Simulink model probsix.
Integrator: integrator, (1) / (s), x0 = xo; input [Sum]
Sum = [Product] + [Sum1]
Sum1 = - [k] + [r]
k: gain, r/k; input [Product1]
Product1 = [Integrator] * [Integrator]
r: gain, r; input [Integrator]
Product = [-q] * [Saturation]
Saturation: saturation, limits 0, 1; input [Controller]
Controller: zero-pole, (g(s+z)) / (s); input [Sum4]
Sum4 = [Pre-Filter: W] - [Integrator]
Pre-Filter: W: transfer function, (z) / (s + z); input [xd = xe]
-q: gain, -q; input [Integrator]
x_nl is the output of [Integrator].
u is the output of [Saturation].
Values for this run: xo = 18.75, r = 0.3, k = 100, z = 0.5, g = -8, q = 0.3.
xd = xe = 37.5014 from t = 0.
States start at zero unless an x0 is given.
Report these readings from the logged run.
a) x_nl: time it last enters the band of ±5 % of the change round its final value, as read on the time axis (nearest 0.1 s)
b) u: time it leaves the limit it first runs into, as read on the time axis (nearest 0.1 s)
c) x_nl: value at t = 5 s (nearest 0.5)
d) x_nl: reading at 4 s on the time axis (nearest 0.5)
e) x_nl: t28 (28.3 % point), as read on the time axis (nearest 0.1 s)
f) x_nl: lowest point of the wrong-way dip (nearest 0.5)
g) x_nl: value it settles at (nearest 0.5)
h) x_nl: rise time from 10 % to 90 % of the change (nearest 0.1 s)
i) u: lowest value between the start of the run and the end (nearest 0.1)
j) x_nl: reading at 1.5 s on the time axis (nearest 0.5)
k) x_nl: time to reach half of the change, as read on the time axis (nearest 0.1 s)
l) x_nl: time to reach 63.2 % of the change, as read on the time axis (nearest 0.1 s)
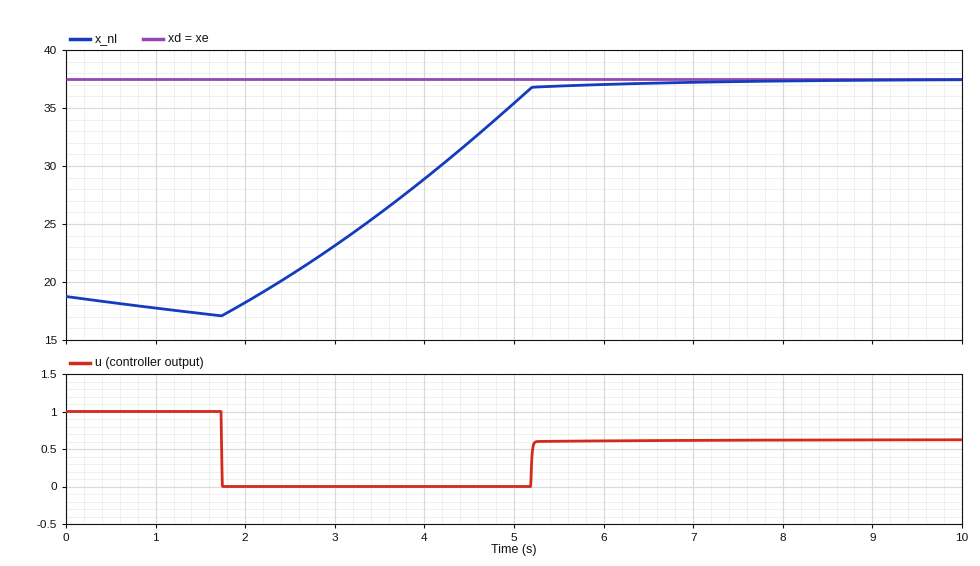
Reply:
5.2 s
1.7 s
35.5
29.0
3.2 s
17.0
37.5
2.5 s
0.0
17.5
3.9 s
4.3 s
